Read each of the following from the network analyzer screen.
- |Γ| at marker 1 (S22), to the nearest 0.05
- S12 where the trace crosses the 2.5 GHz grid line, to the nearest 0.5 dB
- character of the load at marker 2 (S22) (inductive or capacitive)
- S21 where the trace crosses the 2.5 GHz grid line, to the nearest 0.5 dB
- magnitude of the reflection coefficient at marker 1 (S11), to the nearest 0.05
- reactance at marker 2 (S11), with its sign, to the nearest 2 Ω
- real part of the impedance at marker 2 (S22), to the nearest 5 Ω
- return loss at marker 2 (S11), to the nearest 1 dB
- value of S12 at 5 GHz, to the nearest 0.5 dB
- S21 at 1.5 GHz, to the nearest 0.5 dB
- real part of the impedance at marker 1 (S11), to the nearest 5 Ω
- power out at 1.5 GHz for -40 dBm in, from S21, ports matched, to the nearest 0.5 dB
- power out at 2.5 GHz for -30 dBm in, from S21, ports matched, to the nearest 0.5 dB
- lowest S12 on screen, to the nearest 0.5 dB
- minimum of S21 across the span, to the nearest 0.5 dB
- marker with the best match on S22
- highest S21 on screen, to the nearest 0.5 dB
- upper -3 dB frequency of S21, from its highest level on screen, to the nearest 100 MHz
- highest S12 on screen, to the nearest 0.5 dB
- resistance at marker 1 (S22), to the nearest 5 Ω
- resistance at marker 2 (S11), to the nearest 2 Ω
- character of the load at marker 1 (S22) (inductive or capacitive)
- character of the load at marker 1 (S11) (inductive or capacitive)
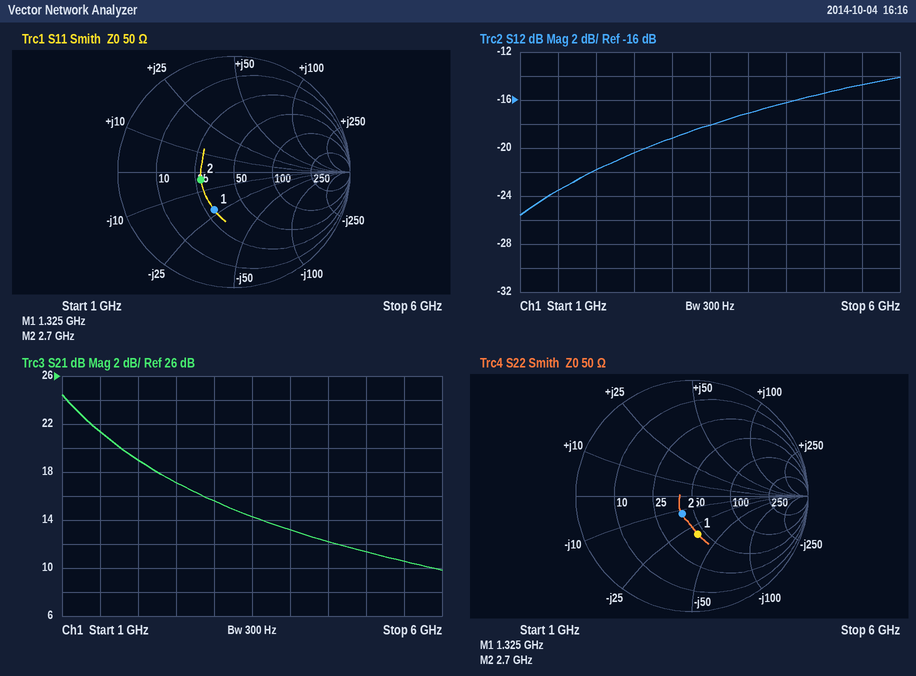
0.35
-20.5 dB
capacitive
17.0 dB
0.35
-4 Ω
40 Ω
11 dB
-15.5 dB
21.5 dB
30 Ω
-18.5 dBm
-13.0 dBm
-25.5 dB
10.0 dB
marker 2
24.5 dB
1.5 GHz
-14.0 dB
45 Ω
28 Ω
capacitive
capacitive
